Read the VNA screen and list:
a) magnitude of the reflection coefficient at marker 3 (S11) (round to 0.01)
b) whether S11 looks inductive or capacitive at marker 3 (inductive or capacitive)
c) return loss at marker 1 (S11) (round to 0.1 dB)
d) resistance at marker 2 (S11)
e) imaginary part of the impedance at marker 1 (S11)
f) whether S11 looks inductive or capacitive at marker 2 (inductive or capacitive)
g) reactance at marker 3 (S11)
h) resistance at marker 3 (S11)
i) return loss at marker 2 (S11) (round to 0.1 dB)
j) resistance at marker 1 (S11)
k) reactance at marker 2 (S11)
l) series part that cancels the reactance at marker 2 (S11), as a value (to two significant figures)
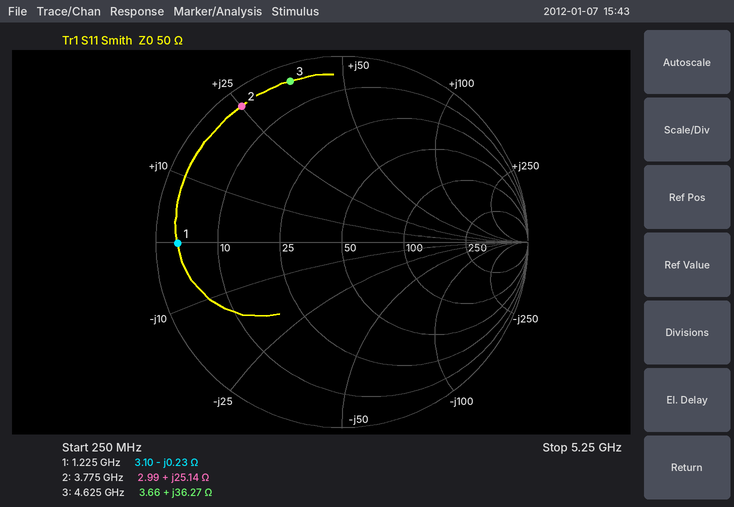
0.91
inductive
1.1 dB
2.99 Ω
-0.23 Ω
inductive
+36.27 Ω
3.66 Ω
0.8 dB
3.10 Ω
+25.14 Ω
1.7 pF
